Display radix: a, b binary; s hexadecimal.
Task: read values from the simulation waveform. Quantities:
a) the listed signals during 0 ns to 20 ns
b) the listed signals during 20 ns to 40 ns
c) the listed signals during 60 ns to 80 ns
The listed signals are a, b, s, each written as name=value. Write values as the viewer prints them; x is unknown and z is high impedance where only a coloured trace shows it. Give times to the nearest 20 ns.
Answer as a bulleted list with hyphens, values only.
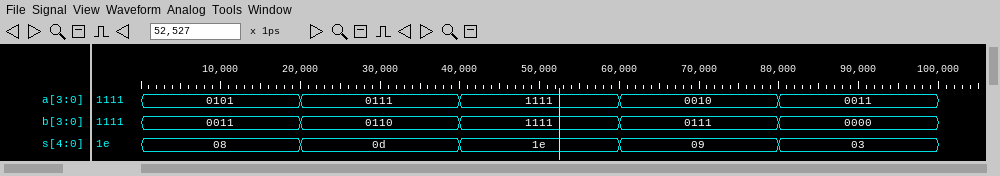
- a=0101, b=0011, s=08
- a=0111, b=0110, s=0d
- a=0010, b=0111, s=09
